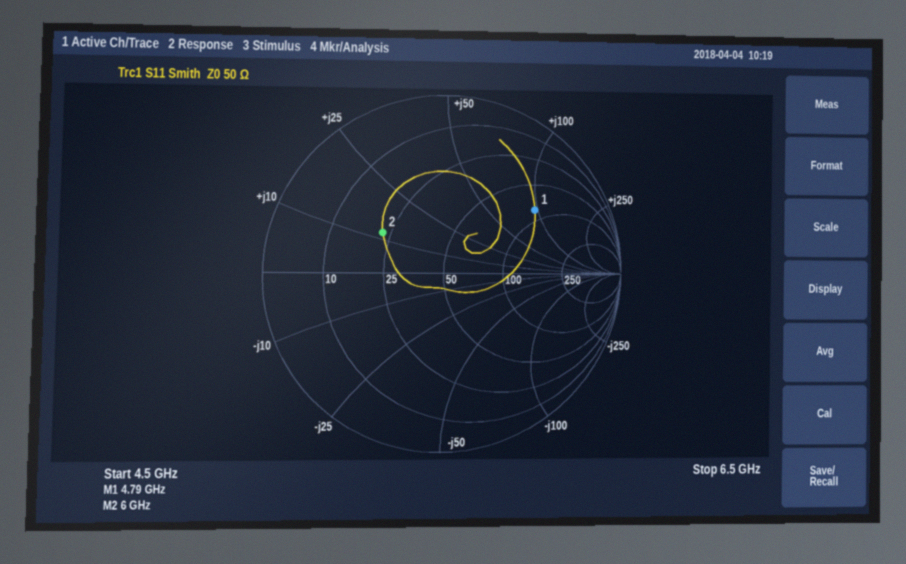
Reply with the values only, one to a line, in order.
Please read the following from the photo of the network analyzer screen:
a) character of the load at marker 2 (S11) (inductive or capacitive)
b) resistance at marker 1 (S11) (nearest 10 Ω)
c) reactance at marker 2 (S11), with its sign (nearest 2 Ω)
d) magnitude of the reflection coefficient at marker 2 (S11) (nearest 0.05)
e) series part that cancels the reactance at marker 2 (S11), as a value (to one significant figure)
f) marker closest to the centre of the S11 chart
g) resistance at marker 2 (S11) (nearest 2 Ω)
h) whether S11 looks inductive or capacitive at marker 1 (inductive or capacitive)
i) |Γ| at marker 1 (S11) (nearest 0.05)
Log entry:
inductive
80 Ω
+12 Ω
0.40
2 pF
marker 2
22 Ω
inductive
0.60
